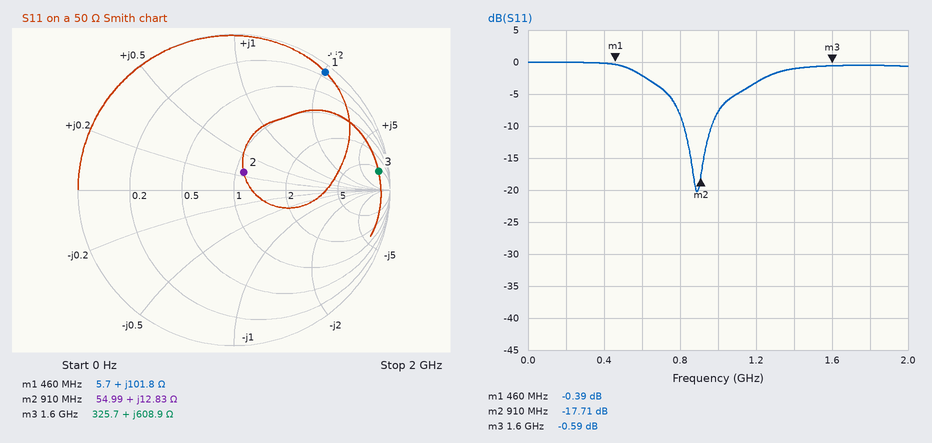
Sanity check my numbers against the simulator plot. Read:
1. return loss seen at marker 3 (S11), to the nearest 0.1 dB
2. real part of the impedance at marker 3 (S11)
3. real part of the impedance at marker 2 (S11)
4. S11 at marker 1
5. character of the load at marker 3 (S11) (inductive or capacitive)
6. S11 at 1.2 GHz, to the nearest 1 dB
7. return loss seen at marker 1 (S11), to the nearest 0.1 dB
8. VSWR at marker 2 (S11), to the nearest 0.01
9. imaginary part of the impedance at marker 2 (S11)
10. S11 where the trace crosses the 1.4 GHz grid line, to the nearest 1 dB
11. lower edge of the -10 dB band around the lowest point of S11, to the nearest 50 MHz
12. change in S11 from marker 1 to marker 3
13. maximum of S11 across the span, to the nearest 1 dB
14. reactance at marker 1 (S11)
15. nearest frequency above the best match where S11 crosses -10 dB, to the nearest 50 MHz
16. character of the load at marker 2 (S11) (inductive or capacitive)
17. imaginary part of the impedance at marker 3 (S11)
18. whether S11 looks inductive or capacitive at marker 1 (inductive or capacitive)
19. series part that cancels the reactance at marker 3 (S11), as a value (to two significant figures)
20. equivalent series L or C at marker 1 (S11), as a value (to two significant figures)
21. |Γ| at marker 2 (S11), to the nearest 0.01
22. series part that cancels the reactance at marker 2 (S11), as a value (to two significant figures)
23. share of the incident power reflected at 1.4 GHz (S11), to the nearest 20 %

0.6 dB
325.7 Ω
54.99 Ω
-0.39 dB
inductive
-3 dB
0.4 dB
1.30
+12.83 Ω
-1 dB
800 MHz
-0.20 dB
0 dB
+101.8 Ω
950 MHz
inductive
+608.9 Ω
inductive
160 fF
35 nH
0.13
14 pF
80 %
